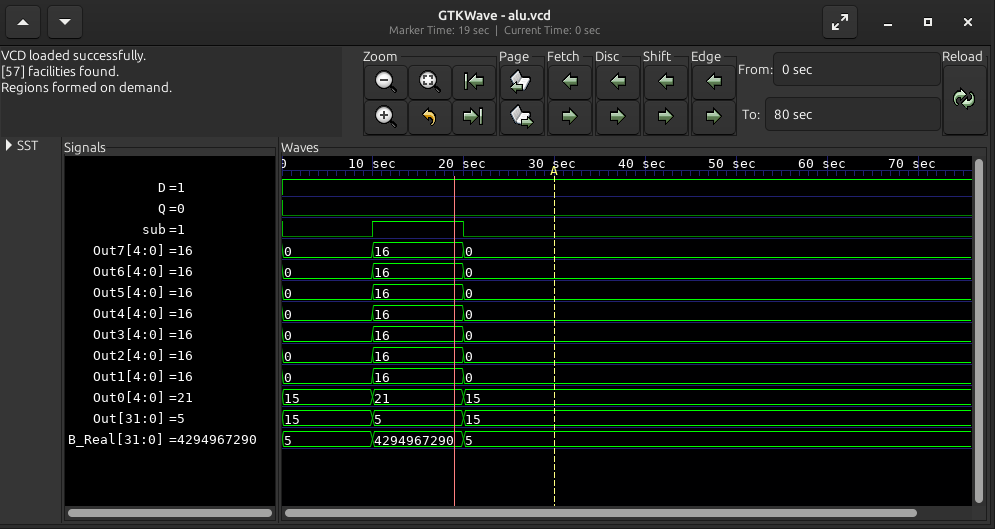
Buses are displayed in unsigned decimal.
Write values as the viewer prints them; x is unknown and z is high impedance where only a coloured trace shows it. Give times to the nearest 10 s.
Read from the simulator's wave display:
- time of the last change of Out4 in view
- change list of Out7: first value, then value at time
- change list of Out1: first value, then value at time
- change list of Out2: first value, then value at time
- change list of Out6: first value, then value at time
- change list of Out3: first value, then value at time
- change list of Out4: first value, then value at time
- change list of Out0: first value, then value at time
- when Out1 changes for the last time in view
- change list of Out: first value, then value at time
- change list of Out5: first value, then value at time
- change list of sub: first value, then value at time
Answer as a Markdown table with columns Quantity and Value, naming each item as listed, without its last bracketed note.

| Quantity | Value |
|---|---|
| time of the last change of Out4 in view | 20 s |
| change list of Out7: first value, then value at time | 0, 16 at 10 s, 0 at 20 s |
| change list of Out1: first value, then value at time | 0, 16 at 10 s, 0 at 20 s |
| change list of Out2: first value, then value at time | 0, 16 at 10 s, 0 at 20 s |
| change list of Out6: first value, then value at time | 0, 16 at 10 s, 0 at 20 s |
| change list of Out3: first value, then value at time | 0, 16 at 10 s, 0 at 20 s |
| change list of Out4: first value, then value at time | 0, 16 at 10 s, 0 at 20 s |
| change list of Out0: first value, then value at time | 15, 21 at 10 s, 15 at 20 s |
| when Out1 changes for the last time in view | 20 s |
| change list of Out: first value, then value at time | 15, 5 at 10 s, 15 at 20 s |
| change list of Out5: first value, then value at time | 0, 16 at 10 s, 0 at 20 s |
| change list of sub: first value, then value at time | 0, 1 at 10 s, 0 at 20 s |
